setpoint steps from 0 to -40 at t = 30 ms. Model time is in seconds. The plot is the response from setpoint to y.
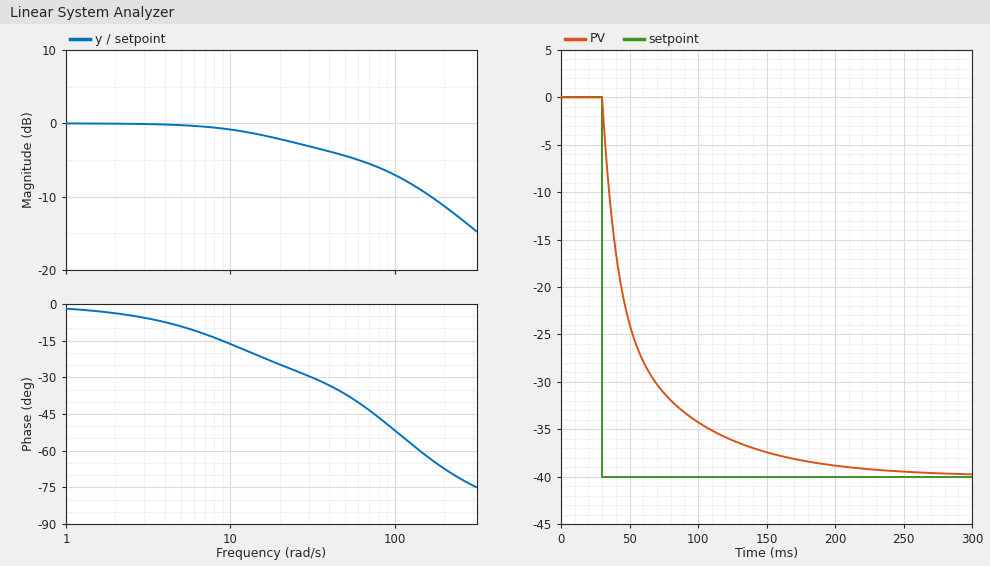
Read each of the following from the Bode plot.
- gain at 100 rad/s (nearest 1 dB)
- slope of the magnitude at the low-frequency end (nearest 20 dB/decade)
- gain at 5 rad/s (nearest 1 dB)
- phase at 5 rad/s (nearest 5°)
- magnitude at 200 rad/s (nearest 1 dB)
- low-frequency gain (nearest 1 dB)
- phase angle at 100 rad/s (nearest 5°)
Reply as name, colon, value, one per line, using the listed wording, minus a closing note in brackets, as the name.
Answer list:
gain at 100 rad/s: -7 dB
slope of the magnitude at the low-frequency end: 0 dB/decade
gain at 5 rad/s: 0 dB
phase at 5 rad/s: -10°
magnitude at 200 rad/s: -11 dB
low-frequency gain: 0 dB
phase angle at 100 rad/s: -50°
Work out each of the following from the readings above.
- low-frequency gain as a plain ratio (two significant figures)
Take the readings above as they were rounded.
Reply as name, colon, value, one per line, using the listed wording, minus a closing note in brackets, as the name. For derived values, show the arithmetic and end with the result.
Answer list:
low-frequency gain as a plain ratio: 10^(0 / 20) = 1.0
